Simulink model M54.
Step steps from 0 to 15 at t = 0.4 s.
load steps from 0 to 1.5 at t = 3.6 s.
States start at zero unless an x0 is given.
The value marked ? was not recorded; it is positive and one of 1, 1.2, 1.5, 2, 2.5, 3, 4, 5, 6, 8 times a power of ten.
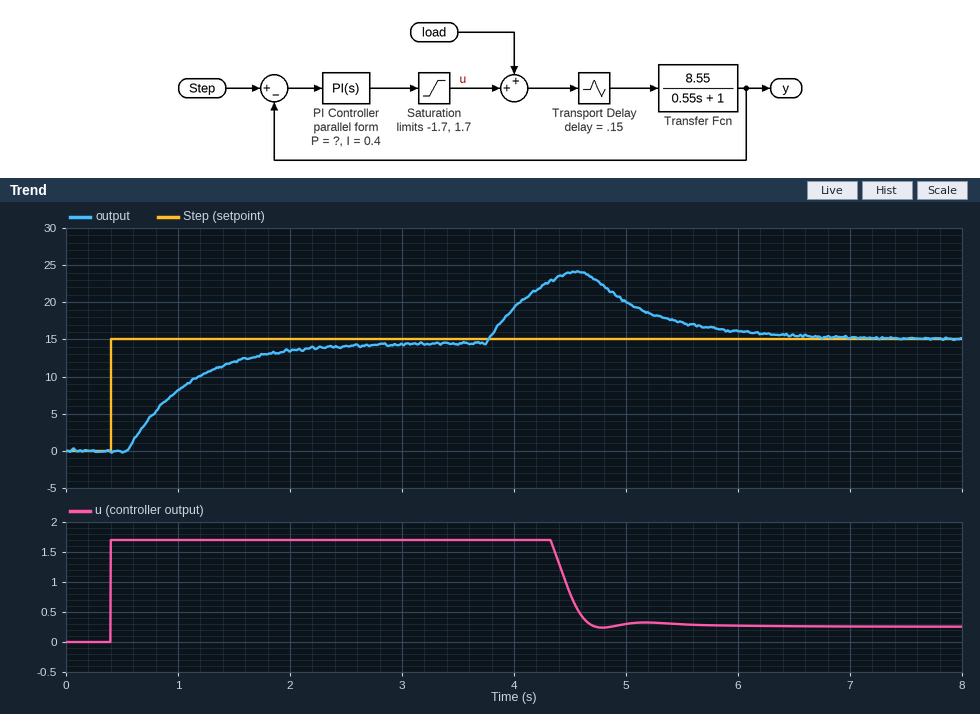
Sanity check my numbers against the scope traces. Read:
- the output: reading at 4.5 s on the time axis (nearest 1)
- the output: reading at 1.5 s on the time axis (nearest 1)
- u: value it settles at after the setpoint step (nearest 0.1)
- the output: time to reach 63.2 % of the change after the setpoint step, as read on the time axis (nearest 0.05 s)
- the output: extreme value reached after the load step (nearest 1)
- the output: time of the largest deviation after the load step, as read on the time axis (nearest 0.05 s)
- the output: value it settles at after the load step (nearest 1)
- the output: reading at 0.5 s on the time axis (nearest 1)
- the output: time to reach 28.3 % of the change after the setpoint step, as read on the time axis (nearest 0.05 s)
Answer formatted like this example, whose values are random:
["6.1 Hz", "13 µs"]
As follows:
["24", "12", "1.7", "1.10 s", "24", "4.55 s", "15", "0", "0.75 s"]
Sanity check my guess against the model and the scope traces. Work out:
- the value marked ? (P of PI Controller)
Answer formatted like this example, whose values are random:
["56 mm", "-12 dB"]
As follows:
["0.25"]
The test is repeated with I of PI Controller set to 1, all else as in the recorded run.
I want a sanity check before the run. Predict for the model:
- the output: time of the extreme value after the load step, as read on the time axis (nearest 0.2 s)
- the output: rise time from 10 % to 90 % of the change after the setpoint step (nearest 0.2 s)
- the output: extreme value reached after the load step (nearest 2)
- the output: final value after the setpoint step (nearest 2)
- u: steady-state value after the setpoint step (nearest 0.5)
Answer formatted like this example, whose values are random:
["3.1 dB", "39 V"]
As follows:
["5.0 s", "1.2 s", "26", "14", "1.5"]
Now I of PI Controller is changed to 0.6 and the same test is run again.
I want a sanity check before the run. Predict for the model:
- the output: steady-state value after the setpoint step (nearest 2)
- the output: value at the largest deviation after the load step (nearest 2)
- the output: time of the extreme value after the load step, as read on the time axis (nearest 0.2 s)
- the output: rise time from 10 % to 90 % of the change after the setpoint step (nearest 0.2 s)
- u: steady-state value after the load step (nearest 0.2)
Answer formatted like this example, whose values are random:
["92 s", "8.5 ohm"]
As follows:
["14", "26", "4.8 s", "1.2 s", "0.2"]
